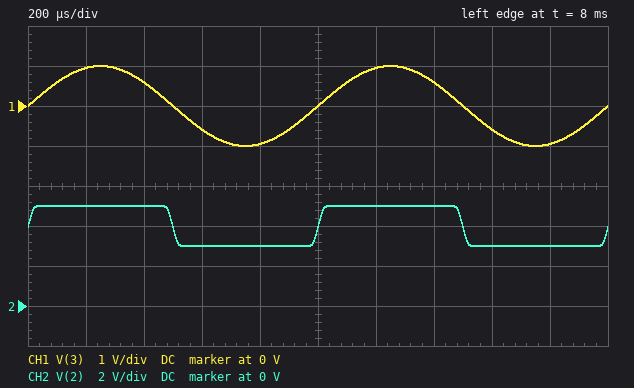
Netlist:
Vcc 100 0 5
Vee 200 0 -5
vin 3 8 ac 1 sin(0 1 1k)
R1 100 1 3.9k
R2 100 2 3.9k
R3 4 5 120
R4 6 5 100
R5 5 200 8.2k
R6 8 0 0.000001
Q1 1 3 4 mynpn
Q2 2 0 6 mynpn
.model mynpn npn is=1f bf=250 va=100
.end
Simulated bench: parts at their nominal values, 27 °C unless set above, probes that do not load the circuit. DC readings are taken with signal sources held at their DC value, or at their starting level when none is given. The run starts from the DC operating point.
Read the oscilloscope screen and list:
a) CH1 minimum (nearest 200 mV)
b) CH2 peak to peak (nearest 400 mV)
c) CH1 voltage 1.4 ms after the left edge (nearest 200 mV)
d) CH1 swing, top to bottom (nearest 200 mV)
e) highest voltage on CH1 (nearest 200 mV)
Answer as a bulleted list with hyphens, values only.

- -1.0 V
- 2.0 V
- 600 mV
- 2.0 V
- 1.0 V
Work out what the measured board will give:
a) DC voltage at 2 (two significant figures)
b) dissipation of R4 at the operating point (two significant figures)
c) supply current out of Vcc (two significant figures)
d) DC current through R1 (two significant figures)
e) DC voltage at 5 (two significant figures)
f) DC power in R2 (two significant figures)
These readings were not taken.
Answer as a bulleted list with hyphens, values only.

- 3.9 V
- 7.5 µW
- 520 µA
- 250 µA
- -710 mV
- 290 µW
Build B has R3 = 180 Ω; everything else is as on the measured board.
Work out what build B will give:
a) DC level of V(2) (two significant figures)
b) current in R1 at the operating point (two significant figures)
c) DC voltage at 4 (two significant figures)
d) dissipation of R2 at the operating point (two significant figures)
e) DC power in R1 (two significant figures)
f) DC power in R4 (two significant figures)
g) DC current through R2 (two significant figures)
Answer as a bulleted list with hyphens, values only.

- 3.8 V
- 220 µA
- -670 mV
- 360 µW
- 180 µW
- 9.3 µW
- 300 µA
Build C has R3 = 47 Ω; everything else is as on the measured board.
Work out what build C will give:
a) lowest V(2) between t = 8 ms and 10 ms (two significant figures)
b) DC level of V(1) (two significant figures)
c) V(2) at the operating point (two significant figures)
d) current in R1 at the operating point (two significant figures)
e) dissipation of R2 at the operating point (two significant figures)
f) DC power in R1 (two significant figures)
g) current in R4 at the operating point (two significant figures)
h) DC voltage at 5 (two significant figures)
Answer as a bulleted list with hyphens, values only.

- 3.0 V
- 3.8 V
- 4.1 V
- 300 µA
- 190 µW
- 350 µW
- 220 µA
- -700 mV
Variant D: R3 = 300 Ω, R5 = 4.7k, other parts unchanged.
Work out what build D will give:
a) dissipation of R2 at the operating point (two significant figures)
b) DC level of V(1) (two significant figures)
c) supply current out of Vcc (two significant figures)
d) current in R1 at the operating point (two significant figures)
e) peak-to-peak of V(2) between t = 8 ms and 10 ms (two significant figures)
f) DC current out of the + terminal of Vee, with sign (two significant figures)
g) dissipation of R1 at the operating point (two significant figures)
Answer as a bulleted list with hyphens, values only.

- 1.5 mW
- 3.9 V
- 900 µA
- 280 µA
- 3.5 V
- -900 µA
- 300 µW
